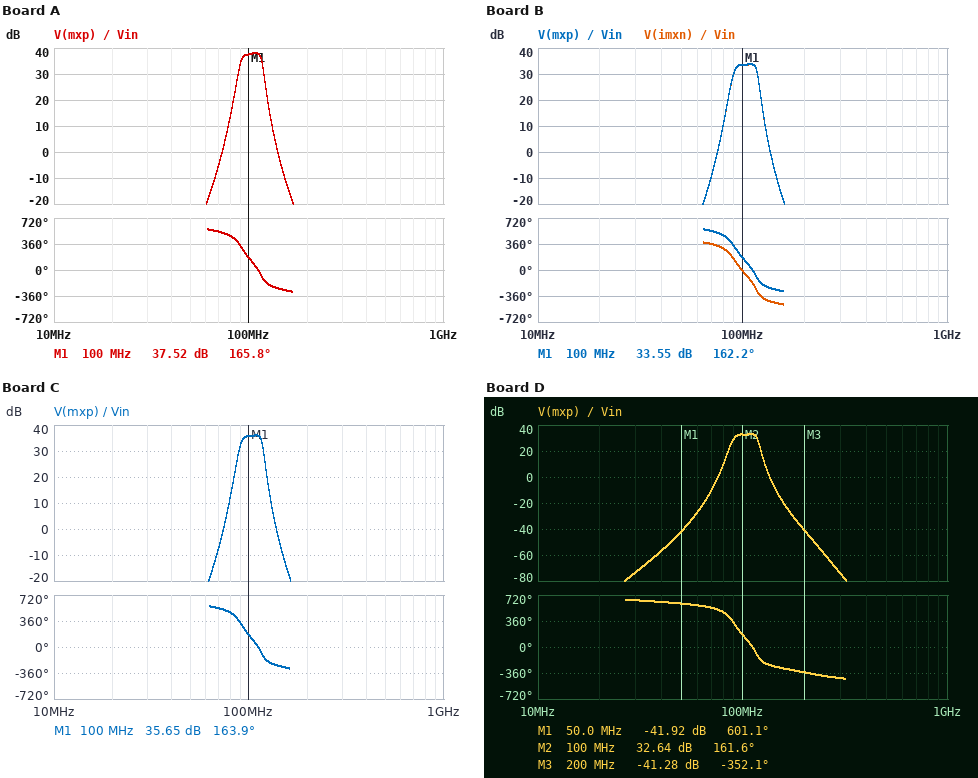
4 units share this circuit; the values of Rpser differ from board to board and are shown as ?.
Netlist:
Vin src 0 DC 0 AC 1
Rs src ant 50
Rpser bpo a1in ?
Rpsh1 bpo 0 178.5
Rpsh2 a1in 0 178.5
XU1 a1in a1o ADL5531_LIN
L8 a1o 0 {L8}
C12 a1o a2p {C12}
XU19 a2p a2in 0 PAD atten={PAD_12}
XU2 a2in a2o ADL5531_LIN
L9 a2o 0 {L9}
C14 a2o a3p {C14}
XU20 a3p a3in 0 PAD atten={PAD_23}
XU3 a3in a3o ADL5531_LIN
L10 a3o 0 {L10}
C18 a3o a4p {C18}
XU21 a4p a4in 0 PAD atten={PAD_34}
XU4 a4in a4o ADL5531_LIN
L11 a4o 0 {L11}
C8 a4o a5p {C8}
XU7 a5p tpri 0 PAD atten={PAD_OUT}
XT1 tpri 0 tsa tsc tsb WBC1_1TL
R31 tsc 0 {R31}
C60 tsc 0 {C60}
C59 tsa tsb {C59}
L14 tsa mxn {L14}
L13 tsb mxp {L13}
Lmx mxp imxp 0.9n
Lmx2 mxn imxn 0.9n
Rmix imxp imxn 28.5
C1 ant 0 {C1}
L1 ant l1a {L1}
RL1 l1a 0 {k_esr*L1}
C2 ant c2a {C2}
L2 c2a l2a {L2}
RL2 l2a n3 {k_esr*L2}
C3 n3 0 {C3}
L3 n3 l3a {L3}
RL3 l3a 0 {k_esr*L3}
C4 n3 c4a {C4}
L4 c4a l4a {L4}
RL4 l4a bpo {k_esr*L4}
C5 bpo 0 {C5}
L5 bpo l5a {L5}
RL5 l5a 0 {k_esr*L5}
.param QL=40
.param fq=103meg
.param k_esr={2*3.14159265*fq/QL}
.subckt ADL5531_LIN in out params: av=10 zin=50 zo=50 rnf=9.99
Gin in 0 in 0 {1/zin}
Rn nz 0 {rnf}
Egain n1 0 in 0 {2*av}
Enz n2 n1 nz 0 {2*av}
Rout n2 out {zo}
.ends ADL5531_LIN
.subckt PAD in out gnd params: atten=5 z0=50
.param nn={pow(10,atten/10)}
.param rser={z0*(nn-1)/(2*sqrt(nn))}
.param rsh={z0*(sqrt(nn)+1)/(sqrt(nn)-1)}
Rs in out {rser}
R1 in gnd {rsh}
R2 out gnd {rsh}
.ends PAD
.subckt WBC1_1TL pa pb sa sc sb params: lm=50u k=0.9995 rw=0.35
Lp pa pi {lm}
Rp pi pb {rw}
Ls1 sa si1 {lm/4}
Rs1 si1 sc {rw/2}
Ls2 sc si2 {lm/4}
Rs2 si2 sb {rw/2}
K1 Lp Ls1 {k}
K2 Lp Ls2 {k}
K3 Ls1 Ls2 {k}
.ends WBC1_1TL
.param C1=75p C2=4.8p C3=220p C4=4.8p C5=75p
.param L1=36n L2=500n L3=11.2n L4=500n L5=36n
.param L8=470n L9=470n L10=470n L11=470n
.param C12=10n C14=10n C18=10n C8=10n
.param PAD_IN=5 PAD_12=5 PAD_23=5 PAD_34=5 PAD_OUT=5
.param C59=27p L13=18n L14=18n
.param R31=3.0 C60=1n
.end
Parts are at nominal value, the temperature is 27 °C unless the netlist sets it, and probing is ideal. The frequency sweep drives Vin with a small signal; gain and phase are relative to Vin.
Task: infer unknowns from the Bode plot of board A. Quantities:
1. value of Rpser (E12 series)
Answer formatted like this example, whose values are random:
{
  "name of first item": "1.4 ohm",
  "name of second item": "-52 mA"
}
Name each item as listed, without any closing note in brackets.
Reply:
{
  "value of Rpser": "22 Ω"
}
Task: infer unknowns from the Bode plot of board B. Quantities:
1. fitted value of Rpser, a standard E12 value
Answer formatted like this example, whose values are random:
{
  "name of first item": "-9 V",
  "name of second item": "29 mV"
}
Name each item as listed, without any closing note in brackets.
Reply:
{
  "fitted value of Rpser, a standard E12 value": "82 Ω"
}
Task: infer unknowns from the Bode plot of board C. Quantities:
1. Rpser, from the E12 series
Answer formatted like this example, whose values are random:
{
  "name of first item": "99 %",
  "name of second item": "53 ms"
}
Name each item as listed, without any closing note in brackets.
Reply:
{
  "Rpser, from the E12 series": "47 Ω"
}
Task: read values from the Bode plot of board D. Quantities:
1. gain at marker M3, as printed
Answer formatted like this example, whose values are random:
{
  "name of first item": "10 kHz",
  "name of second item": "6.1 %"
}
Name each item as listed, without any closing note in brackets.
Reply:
{
  "gain at marker M3, as printed": "-41.28 dB"
}
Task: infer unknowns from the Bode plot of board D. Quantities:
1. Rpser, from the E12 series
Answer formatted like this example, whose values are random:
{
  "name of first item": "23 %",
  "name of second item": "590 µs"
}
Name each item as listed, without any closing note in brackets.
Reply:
{
  "Rpser, from the E12 series": "100 Ω"
}
